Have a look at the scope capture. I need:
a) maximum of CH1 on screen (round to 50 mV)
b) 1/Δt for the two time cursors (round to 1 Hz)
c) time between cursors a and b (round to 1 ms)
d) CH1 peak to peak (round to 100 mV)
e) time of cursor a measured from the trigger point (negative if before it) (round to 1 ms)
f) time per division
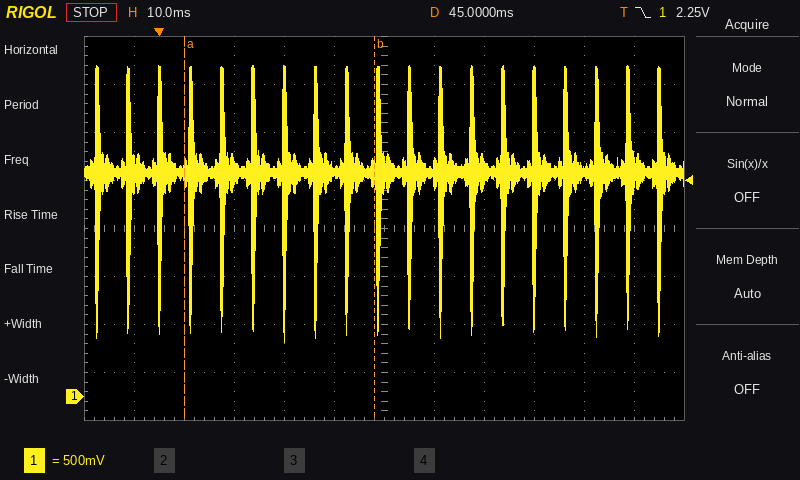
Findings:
3.45 V
26 Hz
38 ms
2.90 V
+5 ms
10 ms
